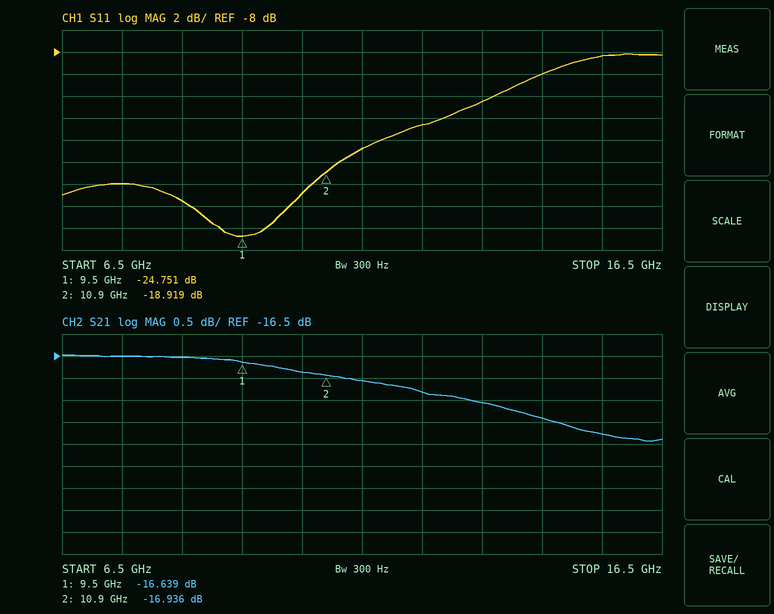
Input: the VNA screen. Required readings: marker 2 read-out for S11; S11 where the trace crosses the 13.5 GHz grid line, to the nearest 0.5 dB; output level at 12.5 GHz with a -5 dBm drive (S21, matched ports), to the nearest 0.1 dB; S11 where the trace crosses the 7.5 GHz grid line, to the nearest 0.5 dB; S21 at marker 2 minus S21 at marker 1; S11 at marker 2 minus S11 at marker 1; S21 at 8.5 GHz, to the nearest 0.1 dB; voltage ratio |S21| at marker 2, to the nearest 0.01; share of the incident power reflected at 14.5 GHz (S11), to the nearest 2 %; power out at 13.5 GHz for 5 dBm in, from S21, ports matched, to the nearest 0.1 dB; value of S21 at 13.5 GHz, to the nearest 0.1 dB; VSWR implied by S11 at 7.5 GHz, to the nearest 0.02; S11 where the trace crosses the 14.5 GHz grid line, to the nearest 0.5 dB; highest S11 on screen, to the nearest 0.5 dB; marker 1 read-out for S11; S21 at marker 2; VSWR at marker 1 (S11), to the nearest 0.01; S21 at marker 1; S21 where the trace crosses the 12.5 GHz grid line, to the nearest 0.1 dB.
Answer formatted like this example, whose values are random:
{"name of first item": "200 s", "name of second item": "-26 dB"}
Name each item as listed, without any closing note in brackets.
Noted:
{"marker 2 read-out for S11": "-18.919 dB", "S11 where the trace crosses the 13.5 GHz grid line, to the nearest 0.5 dB": "-12.5 dB", "output level at 12.5 GHz with a -5 dBm drive (S21, matched ports), to the nearest 0.1 dB": "-22.3 dBm", "S11 where the trace crosses the 7.5 GHz grid line, to the nearest 0.5 dB": "-20.0 dB", "S21 at marker 2 minus S21 at marker 1": "-0.297 dB", "S11 at marker 2 minus S11 at marker 1": "5.832 dB", "S21 at 8.5 GHz, to the nearest 0.1 dB": "-16.5 dB", "voltage ratio |S21| at marker 2, to the nearest 0.01": "0.14", "share of the incident power reflected at 14.5 GHz (S11), to the nearest 2 %": "10 %", "power out at 13.5 GHz for 5 dBm in, from S21, ports matched, to the nearest 0.1 dB": "-12.6 dBm", "value of S21 at 13.5 GHz, to the nearest 0.1 dB": "-17.6 dB", "VSWR implied by S11 at 7.5 GHz, to the nearest 0.02": "1.22", "S11 where the trace crosses the 14.5 GHz grid line, to the nearest 0.5 dB": "-10.0 dB", "highest S11 on screen, to the nearest 0.5 dB": "-8.0 dB", "marker 1 read-out for S11": "-24.751 dB", "S21 at marker 2": "-16.936 dB", "VSWR at marker 1 (S11), to the nearest 0.01": "1.12", "S21 at marker 1": "-16.639 dB", "S21 where the trace crosses the 12.5 GHz grid line, to the nearest 0.1 dB": "-17.3 dB"}
